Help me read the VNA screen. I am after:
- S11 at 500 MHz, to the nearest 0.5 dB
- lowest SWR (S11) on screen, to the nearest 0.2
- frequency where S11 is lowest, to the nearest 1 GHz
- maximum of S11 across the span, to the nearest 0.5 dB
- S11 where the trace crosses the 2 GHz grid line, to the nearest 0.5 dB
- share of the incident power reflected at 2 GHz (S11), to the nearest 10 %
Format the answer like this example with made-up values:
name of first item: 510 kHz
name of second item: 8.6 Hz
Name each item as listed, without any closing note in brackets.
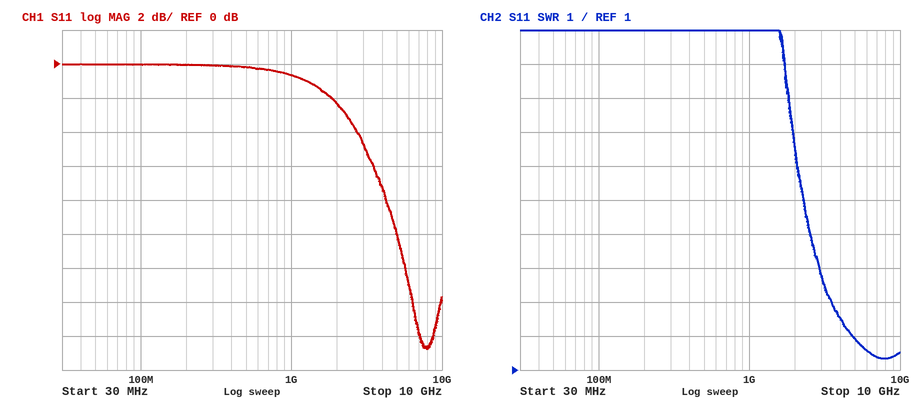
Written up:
S11 at 500 MHz, to the nearest 0.5 dB: 0.0 dB
lowest SWR (S11) on screen, to the nearest 0.2: 1.4
frequency where S11 is lowest, to the nearest 1 GHz: 8 GHz
maximum of S11 across the span, to the nearest 0.5 dB: 0.0 dB
S11 where the trace crosses the 2 GHz grid line, to the nearest 0.5 dB: -2.5 dB
share of the incident power reflected at 2 GHz (S11), to the nearest 10 %: 60 %
